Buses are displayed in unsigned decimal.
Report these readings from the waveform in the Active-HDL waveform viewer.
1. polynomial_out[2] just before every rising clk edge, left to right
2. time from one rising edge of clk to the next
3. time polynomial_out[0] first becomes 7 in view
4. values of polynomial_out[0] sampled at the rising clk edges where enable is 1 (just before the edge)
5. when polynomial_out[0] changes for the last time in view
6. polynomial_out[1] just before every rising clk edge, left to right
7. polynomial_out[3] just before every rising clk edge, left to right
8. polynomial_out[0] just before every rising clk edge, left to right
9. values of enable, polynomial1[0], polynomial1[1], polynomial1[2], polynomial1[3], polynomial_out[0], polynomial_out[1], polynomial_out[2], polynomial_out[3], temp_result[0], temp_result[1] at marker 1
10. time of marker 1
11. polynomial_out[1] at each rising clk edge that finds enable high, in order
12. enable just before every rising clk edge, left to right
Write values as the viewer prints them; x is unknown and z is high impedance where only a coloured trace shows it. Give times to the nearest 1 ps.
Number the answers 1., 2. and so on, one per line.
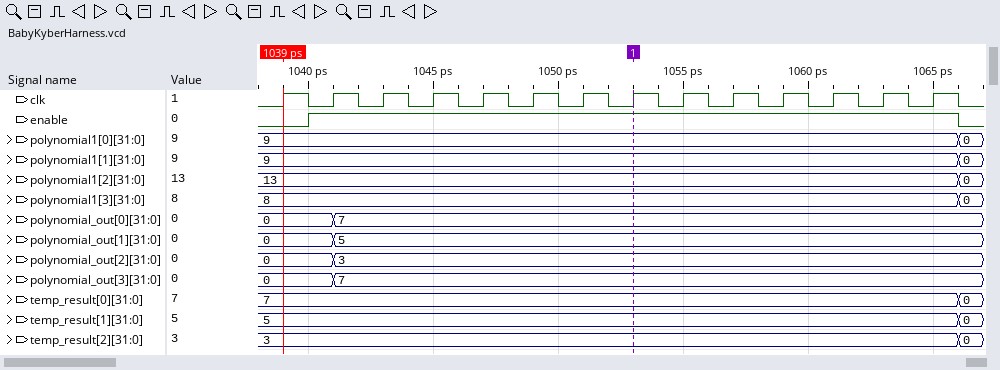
1. 0, 0, 3, 3, 3, 3, 3, 3, 3, 3, 3, 3, 3, 3
2. 2 ps
3. 1041 ps
4. 0, 7, 7, 7, 7, 7, 7, 7, 7, 7, 7, 7, 7
5. 1041 ps
6. 0, 0, 5, 5, 5, 5, 5, 5, 5, 5, 5, 5, 5, 5
7. 0, 0, 7, 7, 7, 7, 7, 7, 7, 7, 7, 7, 7, 7
8. 0, 0, 7, 7, 7, 7, 7, 7, 7, 7, 7, 7, 7, 7
9. enable=1, polynomial1[0]=9, polynomial1[1]=9, polynomial1[2]=13, polynomial1[3]=8, polynomial_out[0]=7, polynomial_out[1]=5, polynomial_out[2]=3, polynomial_out[3]=7, temp_result[0]=7, temp_result[1]=5
10. 1053 ps
11. 0, 5, 5, 5, 5, 5, 5, 5, 5, 5, 5, 5, 5
12. 0 1 1 1 1 1 1 1 1 1 1 1 1 1
